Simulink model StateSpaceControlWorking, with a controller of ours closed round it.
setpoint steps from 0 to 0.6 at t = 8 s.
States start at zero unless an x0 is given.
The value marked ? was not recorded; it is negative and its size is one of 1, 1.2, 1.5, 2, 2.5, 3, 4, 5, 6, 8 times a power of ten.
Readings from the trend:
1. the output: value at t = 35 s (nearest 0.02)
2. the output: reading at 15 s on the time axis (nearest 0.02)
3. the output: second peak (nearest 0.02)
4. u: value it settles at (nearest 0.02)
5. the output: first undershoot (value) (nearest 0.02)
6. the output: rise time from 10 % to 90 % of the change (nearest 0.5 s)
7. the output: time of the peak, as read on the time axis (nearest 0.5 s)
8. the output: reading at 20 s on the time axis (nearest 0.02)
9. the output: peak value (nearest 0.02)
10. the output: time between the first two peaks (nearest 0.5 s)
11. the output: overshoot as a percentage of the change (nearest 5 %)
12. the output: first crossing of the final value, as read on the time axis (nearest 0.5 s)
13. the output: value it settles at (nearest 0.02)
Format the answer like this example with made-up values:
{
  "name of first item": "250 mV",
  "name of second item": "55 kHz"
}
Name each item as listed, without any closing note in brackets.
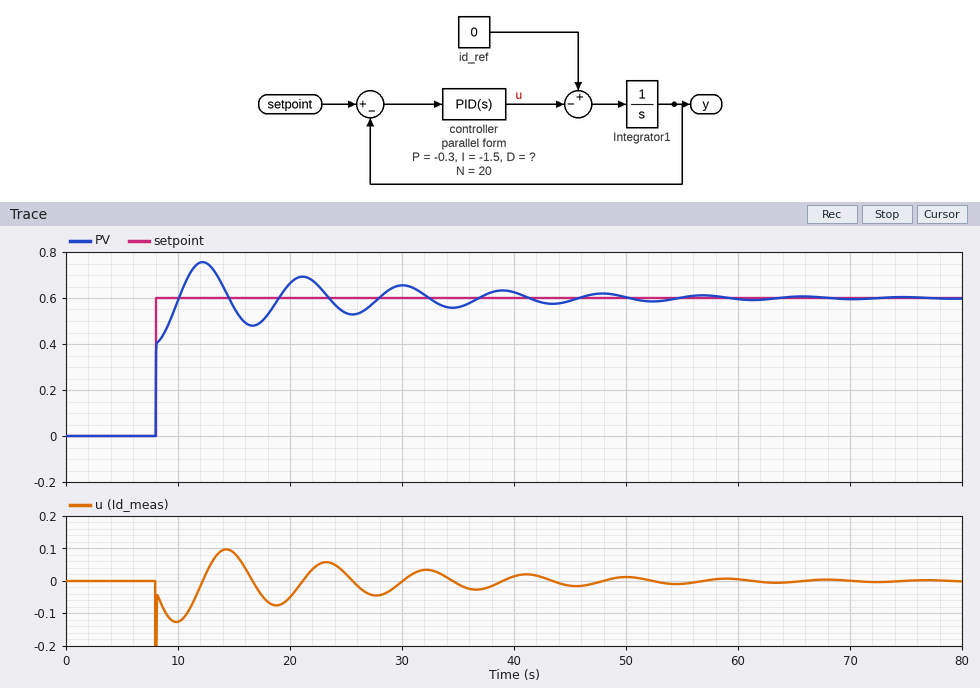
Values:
{
  "the output: value at t = 35 s": "0.56",
  "the output: reading at 15 s on the time axis": "0.56",
  "the output: second peak": "0.70",
  "u: value it settles at": "0.00",
  "the output: first undershoot (value)": "0.48",
  "the output: rise time from 10 % to 90 % of the change": "1.5 s",
  "the output: time of the peak, as read on the time axis": "12.0 s",
  "the output: reading at 20 s on the time axis": "0.66",
  "the output: peak value": "0.76",
  "the output: time between the first two peaks": "9.0 s",
  "the output: overshoot as a percentage of the change": "25 %",
  "the output: first crossing of the final value, as read on the time axis": "10.0 s",
  "the output: value it settles at": "0.60"
}
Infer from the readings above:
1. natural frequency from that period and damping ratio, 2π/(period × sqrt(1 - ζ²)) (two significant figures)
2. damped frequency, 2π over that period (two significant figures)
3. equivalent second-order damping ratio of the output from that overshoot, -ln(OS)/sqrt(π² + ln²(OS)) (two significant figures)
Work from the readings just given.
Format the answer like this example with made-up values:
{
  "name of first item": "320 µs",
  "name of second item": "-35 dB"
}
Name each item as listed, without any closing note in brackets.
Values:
{
  "natural frequency from that period and damping ratio, 2π/(period × sqrt(1 - ζ²))": "0.76 rad/s",
  "damped frequency, 2π over that period": "0.70 rad/s",
  "equivalent second-order damping ratio of the output from that overshoot, -ln(OS)/sqrt(π² + ln²(OS))": "0.40"
}
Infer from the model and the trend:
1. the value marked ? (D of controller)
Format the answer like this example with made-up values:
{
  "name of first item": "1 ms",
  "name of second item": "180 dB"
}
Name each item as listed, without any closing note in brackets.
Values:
{
  "the value marked ?": "-2"
}
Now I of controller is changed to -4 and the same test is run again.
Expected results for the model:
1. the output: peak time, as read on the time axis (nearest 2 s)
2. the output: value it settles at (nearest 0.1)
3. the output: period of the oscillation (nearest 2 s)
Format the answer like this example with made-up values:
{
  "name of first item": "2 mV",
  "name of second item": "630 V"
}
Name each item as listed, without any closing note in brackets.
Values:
{
  "the output: peak time, as read on the time axis": "10 s",
  "the output: value it settles at": "0.6",
  "the output: period of the oscillation": "6 s"
}
